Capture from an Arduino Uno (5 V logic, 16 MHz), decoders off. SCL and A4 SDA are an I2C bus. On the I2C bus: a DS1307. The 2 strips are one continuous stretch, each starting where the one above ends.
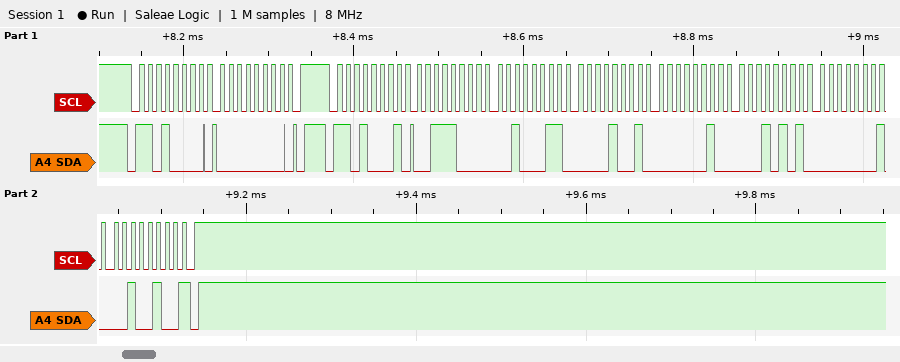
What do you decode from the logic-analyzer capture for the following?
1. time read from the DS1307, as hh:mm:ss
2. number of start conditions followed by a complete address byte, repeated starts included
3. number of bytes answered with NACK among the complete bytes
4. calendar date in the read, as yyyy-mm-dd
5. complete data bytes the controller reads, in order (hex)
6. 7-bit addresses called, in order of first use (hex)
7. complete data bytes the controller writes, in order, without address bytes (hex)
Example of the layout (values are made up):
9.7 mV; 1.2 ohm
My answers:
09:23:38; 2; 1; 2024-01-15; 38 23 09 02 15 01 24; 0x68; 00
